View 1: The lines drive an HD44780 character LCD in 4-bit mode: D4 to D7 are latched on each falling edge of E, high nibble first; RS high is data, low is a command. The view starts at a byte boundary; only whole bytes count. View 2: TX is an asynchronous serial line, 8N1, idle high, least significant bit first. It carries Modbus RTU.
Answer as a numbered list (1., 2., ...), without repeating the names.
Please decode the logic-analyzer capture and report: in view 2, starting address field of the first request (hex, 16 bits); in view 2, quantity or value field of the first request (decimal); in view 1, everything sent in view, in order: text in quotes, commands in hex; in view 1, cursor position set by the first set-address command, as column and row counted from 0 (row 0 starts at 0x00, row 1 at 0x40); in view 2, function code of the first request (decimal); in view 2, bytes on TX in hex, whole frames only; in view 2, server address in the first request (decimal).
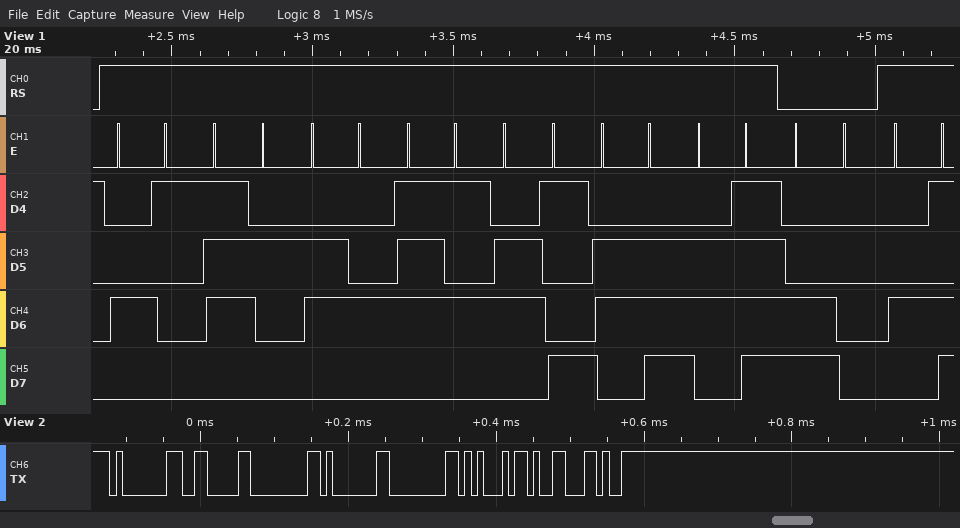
1. 0x0001
2. 69
3. "Arduino" 0xC0 "M"
4. column 0, row 1
5. 6
6. 01 06 00 01 00 45 19 F9
7. 1
